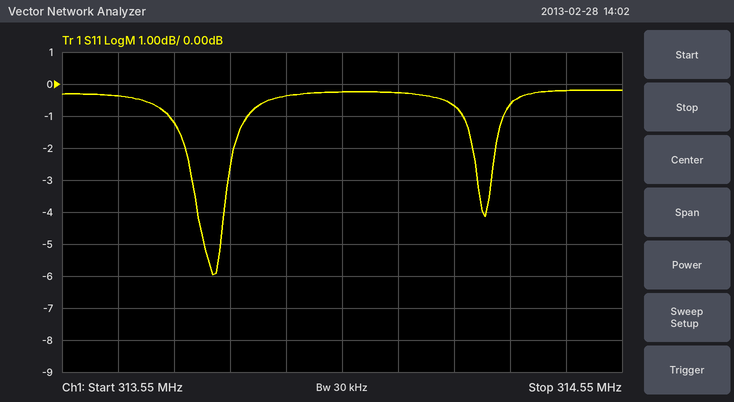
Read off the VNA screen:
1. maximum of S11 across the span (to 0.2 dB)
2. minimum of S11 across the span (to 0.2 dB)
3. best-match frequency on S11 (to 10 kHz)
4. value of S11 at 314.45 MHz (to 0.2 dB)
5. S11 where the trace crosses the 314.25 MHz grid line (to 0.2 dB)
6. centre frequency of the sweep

-0.2 dB
-6.0 dB
313.82 MHz
-0.2 dB
-0.6 dB
314.05 MHz
